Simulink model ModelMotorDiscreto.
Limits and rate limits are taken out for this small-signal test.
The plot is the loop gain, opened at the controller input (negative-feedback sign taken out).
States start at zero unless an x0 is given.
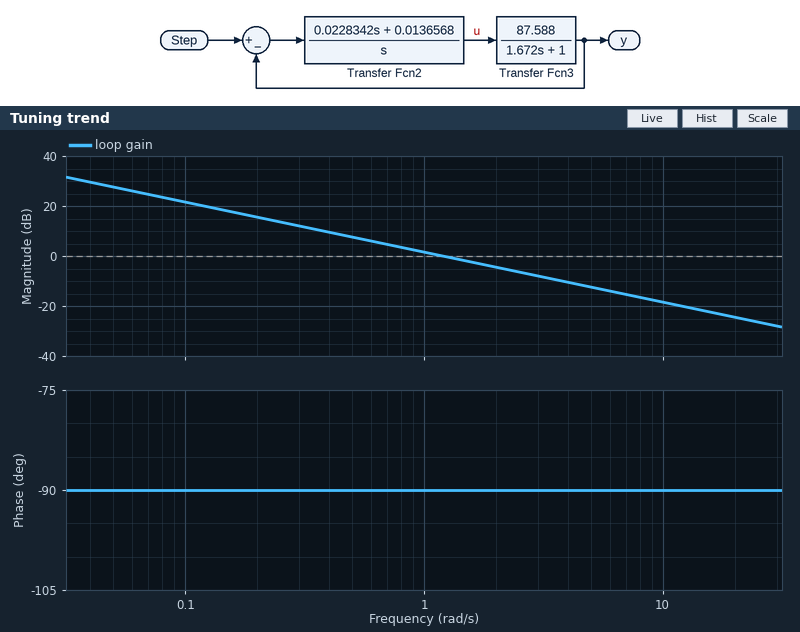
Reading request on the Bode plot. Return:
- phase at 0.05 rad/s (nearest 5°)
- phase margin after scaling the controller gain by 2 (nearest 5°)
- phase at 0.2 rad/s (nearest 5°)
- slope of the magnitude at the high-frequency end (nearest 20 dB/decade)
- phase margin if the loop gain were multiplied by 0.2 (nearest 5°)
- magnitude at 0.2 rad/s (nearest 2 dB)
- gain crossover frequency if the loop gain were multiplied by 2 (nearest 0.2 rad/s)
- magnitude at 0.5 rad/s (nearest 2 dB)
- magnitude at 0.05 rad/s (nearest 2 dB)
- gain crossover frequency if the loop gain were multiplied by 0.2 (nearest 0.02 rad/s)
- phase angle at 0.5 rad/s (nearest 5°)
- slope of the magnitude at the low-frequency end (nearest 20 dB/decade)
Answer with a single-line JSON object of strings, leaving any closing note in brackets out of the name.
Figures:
{"phase at 0.05 rad/s": "-90°", "phase margin after scaling the controller gain by 2": "90°", "phase at 0.2 rad/s": "-90°", "slope of the magnitude at the high-frequency end": "-20 dB/decade", "phase margin if the loop gain were multiplied by 0.2": "90°", "magnitude at 0.2 rad/s": "16 dB", "gain crossover frequency if the loop gain were multiplied by 2": "2.4 rad/s", "magnitude at 0.5 rad/s": "8 dB", "magnitude at 0.05 rad/s": "28 dB", "gain crossover frequency if the loop gain were multiplied by 0.2": "0.24 rad/s", "phase angle at 0.5 rad/s": "-90°", "slope of the magnitude at the low-frequency end": "-20 dB/decade"}
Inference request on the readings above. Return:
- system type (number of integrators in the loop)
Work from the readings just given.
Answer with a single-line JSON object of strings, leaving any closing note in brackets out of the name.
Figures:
{"system type": "1"}
